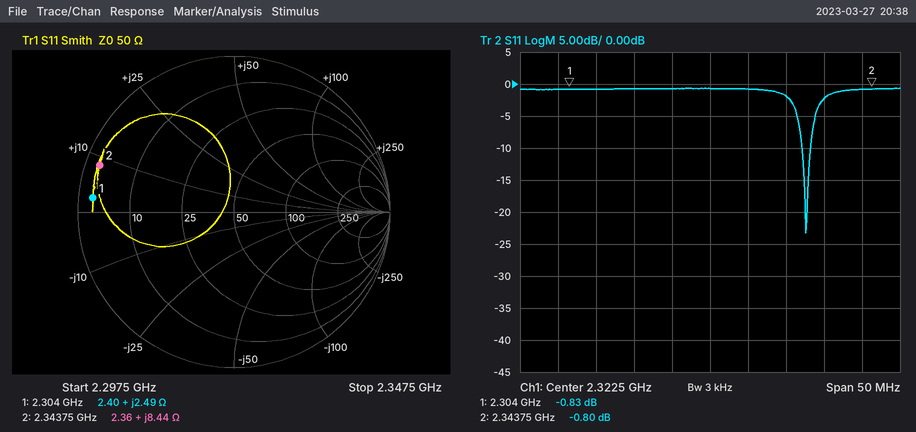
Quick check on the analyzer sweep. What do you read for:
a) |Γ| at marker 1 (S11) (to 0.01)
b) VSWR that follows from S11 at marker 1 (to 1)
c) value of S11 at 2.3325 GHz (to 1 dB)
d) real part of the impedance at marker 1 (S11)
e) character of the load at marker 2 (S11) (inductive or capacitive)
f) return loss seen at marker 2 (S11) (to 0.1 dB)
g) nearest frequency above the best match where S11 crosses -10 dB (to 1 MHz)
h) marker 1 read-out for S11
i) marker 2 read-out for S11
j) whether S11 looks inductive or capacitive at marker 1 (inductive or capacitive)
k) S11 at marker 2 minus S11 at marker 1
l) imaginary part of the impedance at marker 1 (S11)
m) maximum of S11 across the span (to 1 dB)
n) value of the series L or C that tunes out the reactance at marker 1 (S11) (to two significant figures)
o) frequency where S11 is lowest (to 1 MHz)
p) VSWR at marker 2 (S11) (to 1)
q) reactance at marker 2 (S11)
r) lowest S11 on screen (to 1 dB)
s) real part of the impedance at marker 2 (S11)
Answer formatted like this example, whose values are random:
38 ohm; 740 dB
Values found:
0.91; 21; -2 dB; 2.40 Ω; inductive; 0.8 dB; 2.336 GHz; -0.83 dB; -0.80 dB; inductive; 0.03 dB; +2.49 Ω; -1 dB; 28 pF; 2.335 GHz; 22; +8.44 Ω; -23 dB; 2.36 Ω
